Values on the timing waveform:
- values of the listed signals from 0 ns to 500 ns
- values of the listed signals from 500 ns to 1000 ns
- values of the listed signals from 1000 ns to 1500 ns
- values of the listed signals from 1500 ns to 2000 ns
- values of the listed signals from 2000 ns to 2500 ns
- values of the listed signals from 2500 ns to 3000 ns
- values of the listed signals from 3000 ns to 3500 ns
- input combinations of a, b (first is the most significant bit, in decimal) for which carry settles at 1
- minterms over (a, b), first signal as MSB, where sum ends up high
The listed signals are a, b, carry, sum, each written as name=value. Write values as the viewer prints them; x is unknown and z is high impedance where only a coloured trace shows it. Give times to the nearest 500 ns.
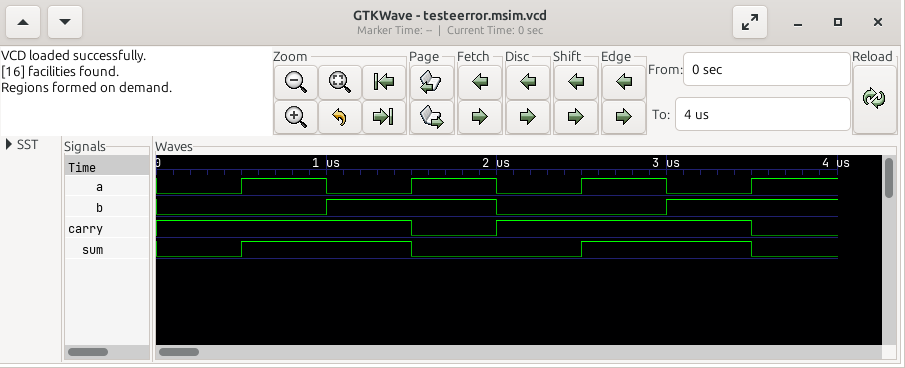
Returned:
a=0, b=0, carry=1, sum=0
a=1, b=0, carry=1, sum=1
a=0, b=1, carry=1, sum=1
a=1, b=1, carry=0, sum=0
a=0, b=0, carry=1, sum=0
a=1, b=0, carry=1, sum=1
a=0, b=1, carry=1, sum=1
0, 1, 2
1, 2
